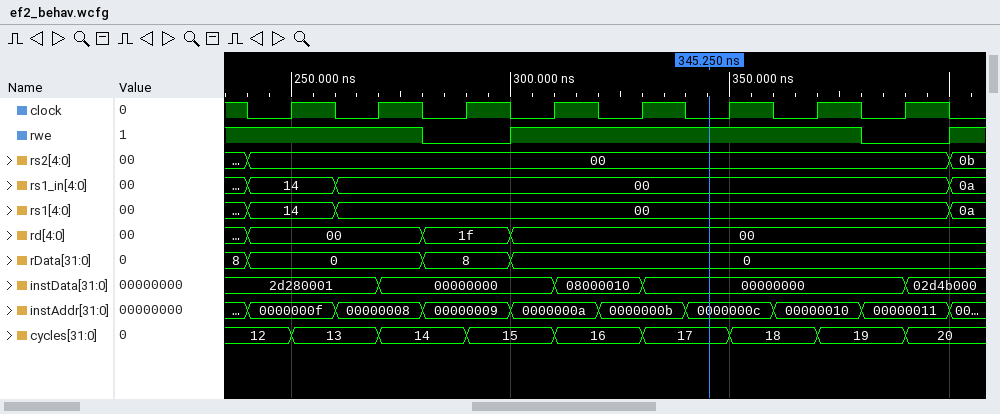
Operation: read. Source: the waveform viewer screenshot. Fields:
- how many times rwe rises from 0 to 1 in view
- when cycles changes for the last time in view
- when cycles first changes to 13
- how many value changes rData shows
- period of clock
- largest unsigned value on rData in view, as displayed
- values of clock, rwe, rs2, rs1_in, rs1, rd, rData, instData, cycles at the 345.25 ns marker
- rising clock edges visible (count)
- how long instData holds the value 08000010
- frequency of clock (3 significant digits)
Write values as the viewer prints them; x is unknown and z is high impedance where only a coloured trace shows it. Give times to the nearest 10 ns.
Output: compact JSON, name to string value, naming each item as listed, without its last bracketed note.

{"how many times rwe rises from 0 to 1 in view": "2", "when cycles changes for the last time in view": "390 ns", "when cycles first changes to 13": "250 ns", "how many value changes rData shows": "3", "period of clock": "20 ns", "largest unsigned value on rData in view, as displayed": "8", "values of clock, rwe, rs2, rs1_in, rs1, rd, rData, instData, cycles at the 345.25 ns marker": "clock=0, rwe=1, rs2=00, rs1_in=00, rs1=00, rd=00, rData=0, instData=00000000, cycles=17", "rising clock edges visible": "8", "how long instData holds the value 08000010": "20 ns", "frequency of clock": "50.0 MHz"}
